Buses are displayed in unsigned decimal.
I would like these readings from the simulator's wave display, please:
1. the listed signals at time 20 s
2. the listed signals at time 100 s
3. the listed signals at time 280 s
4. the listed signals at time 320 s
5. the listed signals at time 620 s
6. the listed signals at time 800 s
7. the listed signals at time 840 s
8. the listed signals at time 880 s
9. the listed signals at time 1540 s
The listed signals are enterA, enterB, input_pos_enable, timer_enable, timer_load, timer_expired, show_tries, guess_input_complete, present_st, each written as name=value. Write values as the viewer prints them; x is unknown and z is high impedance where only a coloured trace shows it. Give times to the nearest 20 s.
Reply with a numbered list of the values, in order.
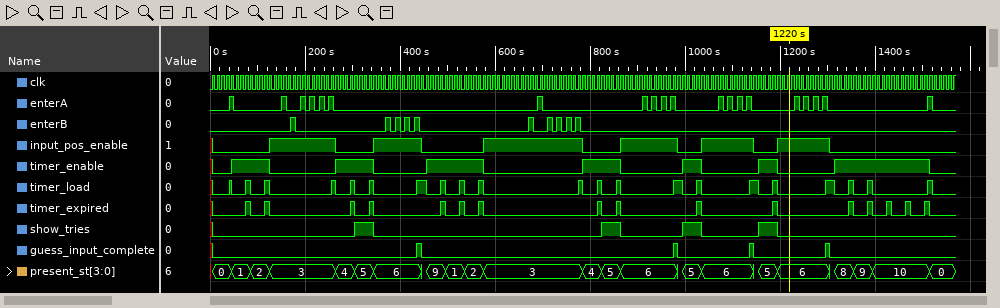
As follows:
1. enterA=0, enterB=0, input_pos_enable=0, timer_enable=0, timer_load=0, timer_expired=0, show_tries=0, guess_input_complete=0, present_st=0
2. enterA=0, enterB=0, input_pos_enable=0, timer_enable=1, timer_load=0, timer_expired=0, show_tries=0, guess_input_complete=0, present_st=2
3. enterA=0, enterB=0, input_pos_enable=0, timer_enable=1, timer_load=0, timer_expired=0, show_tries=0, guess_input_complete=0, present_st=4
4. enterA=0, enterB=0, input_pos_enable=0, timer_enable=1, timer_load=0, timer_expired=0, show_tries=1, guess_input_complete=0, present_st=5
5. enterA=0, enterB=0, input_pos_enable=1, timer_enable=0, timer_load=0, timer_expired=0, show_tries=0, guess_input_complete=0, present_st=3
6. enterA=0, enterB=0, input_pos_enable=0, timer_enable=1, timer_load=0, timer_expired=0, show_tries=0, guess_input_complete=0, present_st=4
7. enterA=0, enterB=0, input_pos_enable=0, timer_enable=1, timer_load=0, timer_expired=0, show_tries=1, guess_input_complete=0, present_st=5
8. enterA=0, enterB=0, input_pos_enable=1, timer_enable=0, timer_load=0, timer_expired=0, show_tries=0, guess_input_complete=0, present_st=6
9. enterA=0, enterB=0, input_pos_enable=0, timer_enable=0, timer_load=0, timer_expired=0, show_tries=0, guess_input_complete=0, present_st=0
